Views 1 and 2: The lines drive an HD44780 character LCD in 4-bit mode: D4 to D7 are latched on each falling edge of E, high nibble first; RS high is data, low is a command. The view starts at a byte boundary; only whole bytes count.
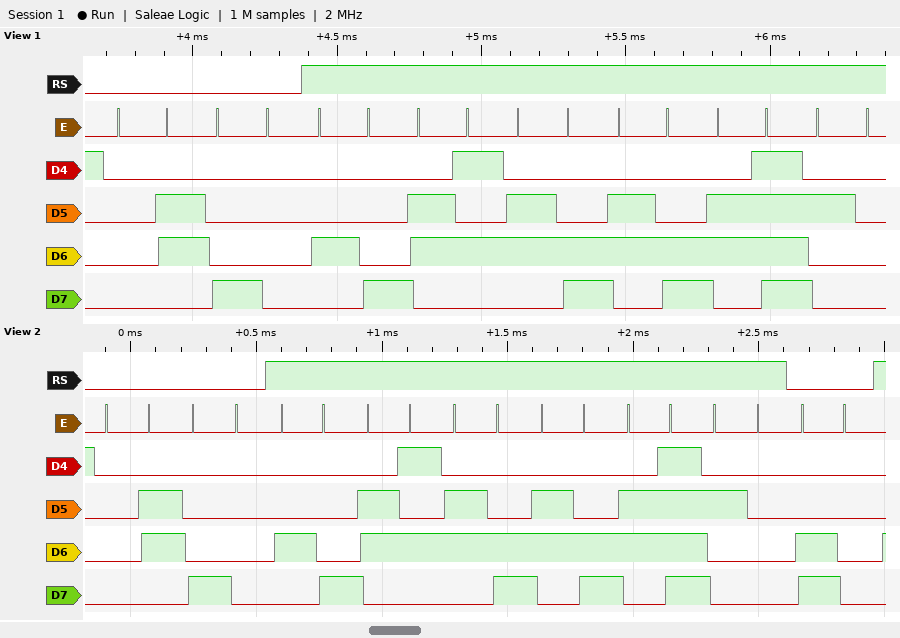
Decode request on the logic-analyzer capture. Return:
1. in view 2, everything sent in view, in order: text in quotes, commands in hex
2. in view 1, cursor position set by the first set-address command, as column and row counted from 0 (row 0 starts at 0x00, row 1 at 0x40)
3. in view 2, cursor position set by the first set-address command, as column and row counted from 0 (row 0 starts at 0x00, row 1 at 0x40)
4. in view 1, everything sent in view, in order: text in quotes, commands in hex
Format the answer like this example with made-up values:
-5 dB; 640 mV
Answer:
0x06 0x80 "Hello " 0xC0; column 0, row 0; column 0, row 0; 0x06 0x80 "Hello "
